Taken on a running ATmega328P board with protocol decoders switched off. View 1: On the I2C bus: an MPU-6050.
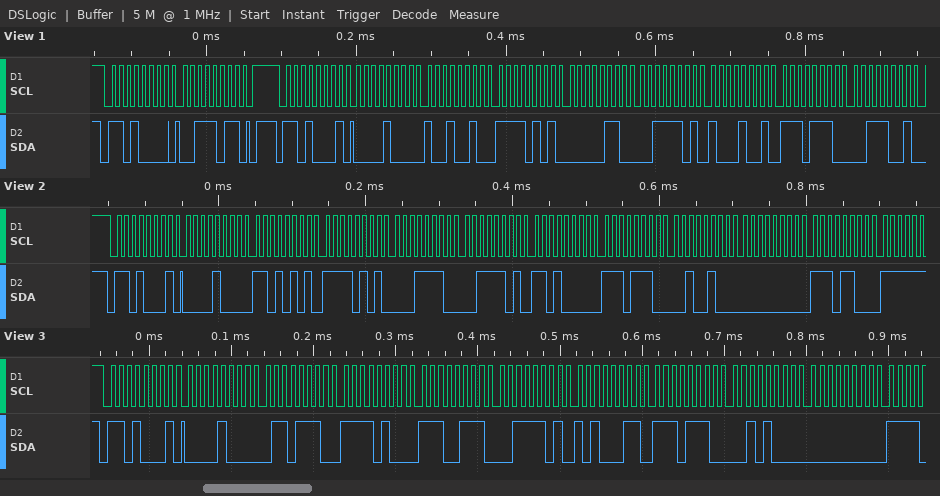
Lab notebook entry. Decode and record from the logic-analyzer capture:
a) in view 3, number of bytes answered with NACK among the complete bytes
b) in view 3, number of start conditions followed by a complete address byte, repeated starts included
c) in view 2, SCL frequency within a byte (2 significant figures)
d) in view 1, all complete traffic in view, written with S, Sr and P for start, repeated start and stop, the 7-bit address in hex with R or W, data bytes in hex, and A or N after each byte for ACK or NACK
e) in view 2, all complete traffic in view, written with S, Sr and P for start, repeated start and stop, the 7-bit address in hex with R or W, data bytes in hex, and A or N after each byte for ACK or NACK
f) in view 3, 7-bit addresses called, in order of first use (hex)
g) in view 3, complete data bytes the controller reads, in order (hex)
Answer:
0
1
100 kHz
S 68W A 3B A P S 68R A 08 A 92 A F5 A 06 A 3D A 89 A EE A 39 A
S 68R A 08 A D5 A F5 A 1E A 3D A D0 A EE A 24 A 00 A EC A
0x68
08 6E F4 E7 3D A3 EE 28 00
